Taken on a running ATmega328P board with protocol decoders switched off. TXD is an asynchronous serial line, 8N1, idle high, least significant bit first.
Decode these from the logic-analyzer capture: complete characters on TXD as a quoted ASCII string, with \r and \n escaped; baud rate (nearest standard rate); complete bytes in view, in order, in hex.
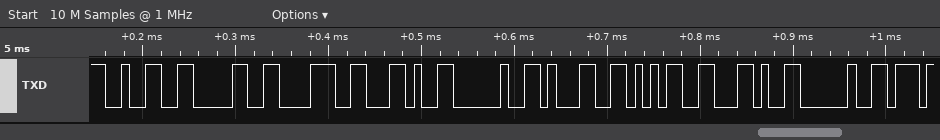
"208, 15, "
115200 baud
0x32 0x30 0x38 0x2C 0x20 0x31 0x35 0x2C 0x20
